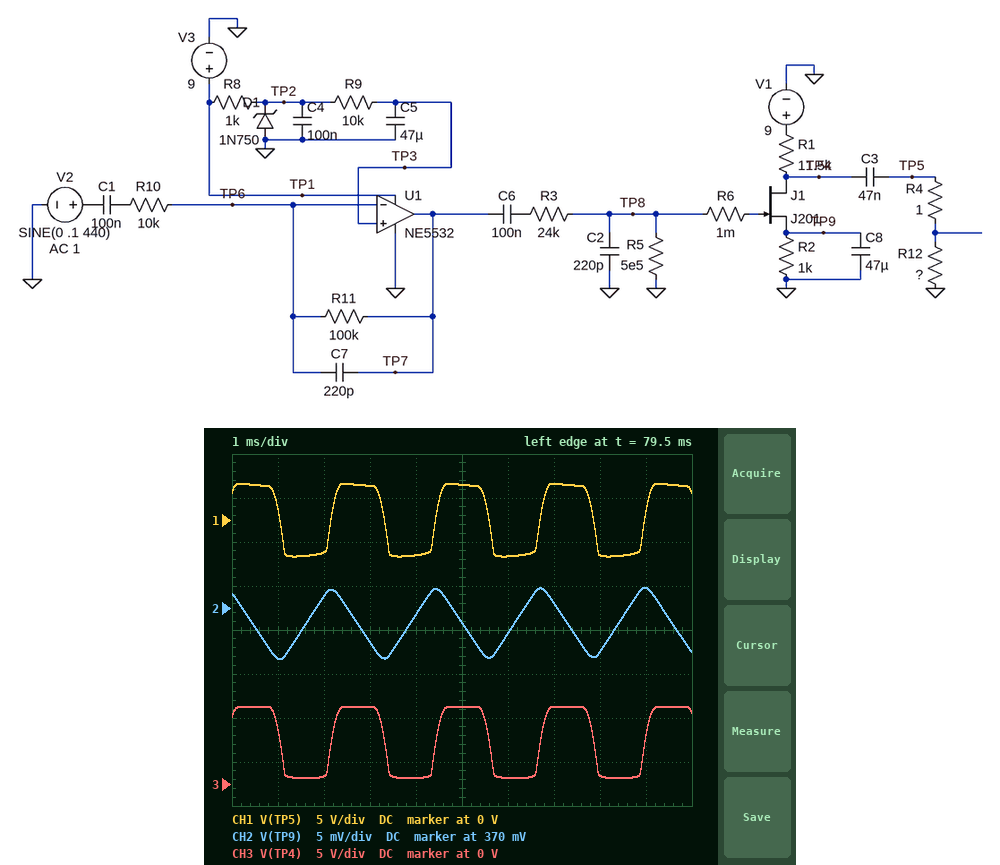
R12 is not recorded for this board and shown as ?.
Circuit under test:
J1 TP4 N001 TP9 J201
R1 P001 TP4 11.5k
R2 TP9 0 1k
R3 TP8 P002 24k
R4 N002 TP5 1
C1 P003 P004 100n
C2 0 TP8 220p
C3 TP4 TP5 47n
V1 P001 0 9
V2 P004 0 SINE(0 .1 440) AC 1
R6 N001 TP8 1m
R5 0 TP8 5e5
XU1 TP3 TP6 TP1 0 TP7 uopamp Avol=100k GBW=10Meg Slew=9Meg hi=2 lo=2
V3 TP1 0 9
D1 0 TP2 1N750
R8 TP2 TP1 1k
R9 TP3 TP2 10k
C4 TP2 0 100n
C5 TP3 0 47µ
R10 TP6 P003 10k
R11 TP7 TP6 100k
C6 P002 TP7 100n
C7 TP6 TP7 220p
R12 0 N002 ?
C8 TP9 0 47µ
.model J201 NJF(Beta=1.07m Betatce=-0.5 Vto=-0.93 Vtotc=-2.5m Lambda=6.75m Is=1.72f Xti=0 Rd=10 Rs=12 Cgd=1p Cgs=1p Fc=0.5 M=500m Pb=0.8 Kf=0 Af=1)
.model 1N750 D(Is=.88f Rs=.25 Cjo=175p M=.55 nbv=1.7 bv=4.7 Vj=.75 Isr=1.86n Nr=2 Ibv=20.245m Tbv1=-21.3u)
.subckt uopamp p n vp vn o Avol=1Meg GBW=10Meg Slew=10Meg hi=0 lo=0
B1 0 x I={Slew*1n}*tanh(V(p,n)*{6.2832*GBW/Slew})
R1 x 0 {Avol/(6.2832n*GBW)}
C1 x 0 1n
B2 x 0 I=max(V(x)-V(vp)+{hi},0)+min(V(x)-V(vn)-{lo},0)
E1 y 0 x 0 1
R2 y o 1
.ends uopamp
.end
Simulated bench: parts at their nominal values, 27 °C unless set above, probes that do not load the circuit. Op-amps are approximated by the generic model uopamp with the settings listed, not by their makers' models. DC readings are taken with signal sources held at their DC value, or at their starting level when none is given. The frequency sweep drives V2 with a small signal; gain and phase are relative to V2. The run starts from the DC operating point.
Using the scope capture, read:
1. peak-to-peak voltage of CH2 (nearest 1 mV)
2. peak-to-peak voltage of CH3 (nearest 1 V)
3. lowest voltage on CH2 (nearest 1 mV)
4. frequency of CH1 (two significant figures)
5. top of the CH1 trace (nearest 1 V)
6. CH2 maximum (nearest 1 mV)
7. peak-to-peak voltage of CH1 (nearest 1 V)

8 mV
8 V
364 mV
440 Hz
4 V
372 mV
8 V
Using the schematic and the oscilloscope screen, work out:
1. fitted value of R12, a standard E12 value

180 kΩ
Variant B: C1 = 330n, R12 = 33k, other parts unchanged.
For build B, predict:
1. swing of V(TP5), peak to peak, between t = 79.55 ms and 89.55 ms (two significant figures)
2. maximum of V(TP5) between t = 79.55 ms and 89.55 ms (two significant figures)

8.2 V
3.8 V
